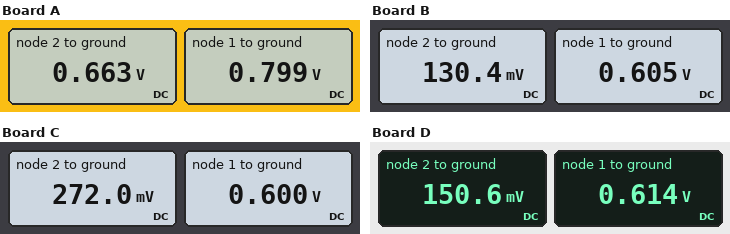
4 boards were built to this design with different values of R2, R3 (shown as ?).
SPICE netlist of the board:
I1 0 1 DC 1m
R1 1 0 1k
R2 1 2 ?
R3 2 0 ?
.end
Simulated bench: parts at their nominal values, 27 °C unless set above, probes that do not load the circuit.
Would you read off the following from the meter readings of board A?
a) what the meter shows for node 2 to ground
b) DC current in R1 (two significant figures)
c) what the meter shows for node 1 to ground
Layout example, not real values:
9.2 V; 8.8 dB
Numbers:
0.663 V; 800 µA; 0.799 V
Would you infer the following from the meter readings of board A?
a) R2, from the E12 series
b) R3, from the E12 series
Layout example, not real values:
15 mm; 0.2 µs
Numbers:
680 Ω; 3.3 kΩ
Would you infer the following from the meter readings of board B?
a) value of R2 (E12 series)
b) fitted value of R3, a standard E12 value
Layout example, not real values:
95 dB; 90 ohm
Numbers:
1.2 kΩ; 330 Ω
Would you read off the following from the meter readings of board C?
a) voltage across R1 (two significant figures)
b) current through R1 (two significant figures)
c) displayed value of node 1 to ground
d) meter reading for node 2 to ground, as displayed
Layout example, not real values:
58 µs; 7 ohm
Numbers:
600 mV; 600 µA; 0.600 V; 272.0 mV
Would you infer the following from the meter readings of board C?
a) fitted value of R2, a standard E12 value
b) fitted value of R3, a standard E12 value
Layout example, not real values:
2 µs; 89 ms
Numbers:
820 Ω; 680 Ω
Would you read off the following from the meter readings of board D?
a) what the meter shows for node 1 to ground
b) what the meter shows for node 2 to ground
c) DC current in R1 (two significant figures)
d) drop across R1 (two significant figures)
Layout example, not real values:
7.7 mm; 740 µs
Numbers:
0.614 V; 150.6 mV; 610 µA; 610 mV
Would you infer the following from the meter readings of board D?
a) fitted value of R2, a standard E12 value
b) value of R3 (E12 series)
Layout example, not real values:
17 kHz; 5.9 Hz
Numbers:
1.2 kΩ; 390 Ω
